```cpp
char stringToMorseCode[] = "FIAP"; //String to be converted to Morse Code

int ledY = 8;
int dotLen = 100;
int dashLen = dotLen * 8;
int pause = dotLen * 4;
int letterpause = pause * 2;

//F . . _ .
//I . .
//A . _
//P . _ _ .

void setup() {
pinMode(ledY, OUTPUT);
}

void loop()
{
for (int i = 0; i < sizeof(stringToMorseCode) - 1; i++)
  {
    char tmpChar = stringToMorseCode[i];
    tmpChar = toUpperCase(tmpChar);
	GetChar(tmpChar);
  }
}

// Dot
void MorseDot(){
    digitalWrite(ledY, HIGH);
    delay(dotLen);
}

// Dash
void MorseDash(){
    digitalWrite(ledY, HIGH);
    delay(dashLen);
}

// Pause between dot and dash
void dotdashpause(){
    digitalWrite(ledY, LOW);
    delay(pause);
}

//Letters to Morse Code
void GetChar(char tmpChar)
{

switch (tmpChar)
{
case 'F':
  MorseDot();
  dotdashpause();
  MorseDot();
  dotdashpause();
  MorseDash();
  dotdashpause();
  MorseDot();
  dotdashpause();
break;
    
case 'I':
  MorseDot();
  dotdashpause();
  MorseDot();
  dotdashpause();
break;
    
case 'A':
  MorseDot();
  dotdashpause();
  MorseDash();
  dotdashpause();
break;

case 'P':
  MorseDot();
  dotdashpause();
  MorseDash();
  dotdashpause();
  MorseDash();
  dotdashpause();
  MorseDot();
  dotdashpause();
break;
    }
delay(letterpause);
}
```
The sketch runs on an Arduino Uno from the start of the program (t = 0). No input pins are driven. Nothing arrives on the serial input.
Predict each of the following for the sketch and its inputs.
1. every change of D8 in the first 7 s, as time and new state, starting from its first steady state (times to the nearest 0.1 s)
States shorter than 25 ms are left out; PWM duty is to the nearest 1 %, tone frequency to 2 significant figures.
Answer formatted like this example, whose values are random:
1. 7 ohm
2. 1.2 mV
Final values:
1. 0 s high; 0.1 s low; 0.5 s high; 0.6 s low; 1 s high; 1.8 s low; 2.2 s high; 2.3 s low; 3.5 s high; 3.6 s low; 4 s high; 4.1 s low; 5.3 s high; 5.4 s low; 5.8 s high; 6.6 s low
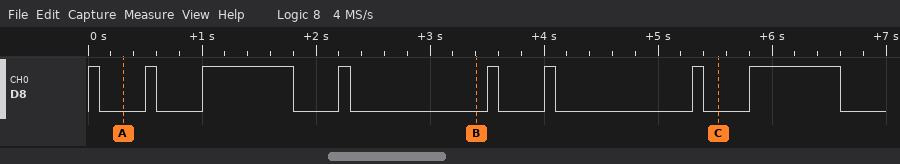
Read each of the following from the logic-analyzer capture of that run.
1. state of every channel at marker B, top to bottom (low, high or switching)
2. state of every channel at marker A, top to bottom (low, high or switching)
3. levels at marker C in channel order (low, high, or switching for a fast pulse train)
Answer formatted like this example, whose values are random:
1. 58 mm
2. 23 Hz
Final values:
1. D8 low
2. D8 low
3. D8 low
